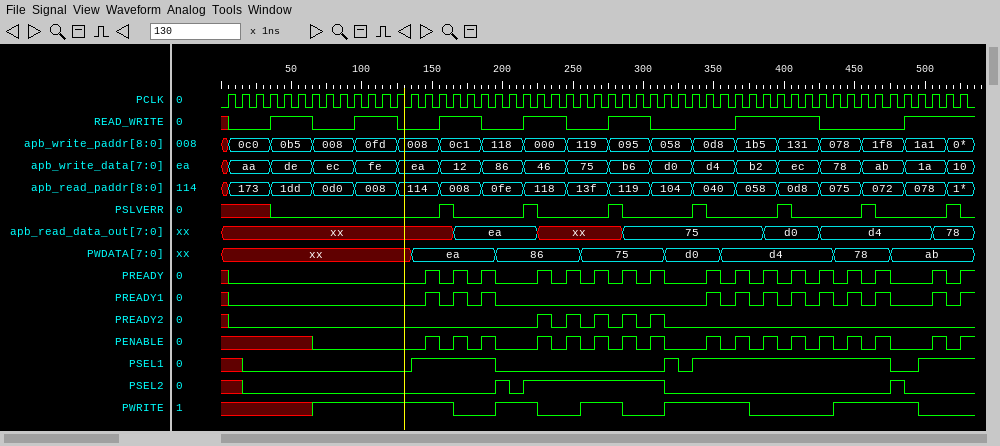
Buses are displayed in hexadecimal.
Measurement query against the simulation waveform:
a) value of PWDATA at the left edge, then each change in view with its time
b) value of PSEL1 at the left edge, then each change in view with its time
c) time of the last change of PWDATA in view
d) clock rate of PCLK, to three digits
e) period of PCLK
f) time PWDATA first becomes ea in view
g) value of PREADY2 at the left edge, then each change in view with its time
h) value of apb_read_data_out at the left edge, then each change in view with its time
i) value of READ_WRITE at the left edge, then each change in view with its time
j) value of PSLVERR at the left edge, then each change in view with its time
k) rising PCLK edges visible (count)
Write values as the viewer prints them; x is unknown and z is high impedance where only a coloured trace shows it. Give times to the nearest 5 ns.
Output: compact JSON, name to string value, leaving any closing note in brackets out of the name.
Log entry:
{"value of PWDATA at the left edge, then each change in view with its time": "xx, ea at 135 ns, 86 at 195 ns, 75 at 255 ns, d0 at 315 ns, d4 at 355 ns, 78 at 435 ns, ab at 475 ns", "value of PSEL1 at the left edge, then each change in view with its time": "x, 0 at 15 ns, 1 at 135 ns, 0 at 195 ns, 1 at 315 ns, 0 at 325 ns, 1 at 335 ns, 0 at 475 ns, 1 at 495 ns", "time of the last change of PWDATA in view": "475 ns", "clock rate of PCLK, to three digits": "100 MHz", "period of PCLK": "10 ns", "time PWDATA first becomes ea in view": "135 ns", "value of PREADY2 at the left edge, then each change in view with its time": "x, 0 at 5 ns, 1 at 225 ns, 0 at 235 ns, 1 at 245 ns, 0 at 255 ns, 1 at 265 ns, 0 at 275 ns, 1 at 285 ns, 0 at 295 ns, 1 at 305 ns, 0 at 315 ns", "value of apb_read_data_out at the left edge, then each change in view with its time": "xx, ea at 165 ns, xx at 225 ns, 75 at 285 ns, d0 at 385 ns, d4 at 425 ns, 78 at 505 ns", "value of READ_WRITE at the left edge, then each change in view with its time": "x, 0 at 5 ns, 1 at 35 ns, 0 at 65 ns, 1 at 95 ns, 0 at 125 ns, 1 at 155 ns, 0 at 185 ns, 1 at 215 ns, 0 at 245 ns, 1 at 275 ns, 0 at 305 ns, 1 at 365 ns, 0 at 425 ns, 1 at 485 ns", "value of PSLVERR at the left edge, then each change in view with its time": "x, 0 at 35 ns, 1 at 155 ns, 0 at 165 ns, 1 at 215 ns, 0 at 225 ns, 1 at 275 ns, 0 at 285 ns, 1 at 335 ns, 0 at 345 ns, 1 at 395 ns, 0 at 405 ns, 1 at 455 ns, 0 at 465 ns, 1 at 515 ns, 0 at 525 ns", "rising PCLK edges visible": "53"}
